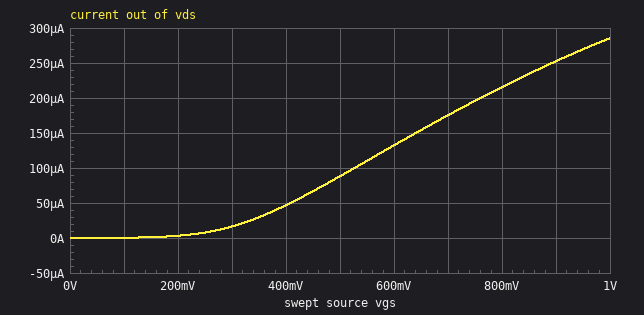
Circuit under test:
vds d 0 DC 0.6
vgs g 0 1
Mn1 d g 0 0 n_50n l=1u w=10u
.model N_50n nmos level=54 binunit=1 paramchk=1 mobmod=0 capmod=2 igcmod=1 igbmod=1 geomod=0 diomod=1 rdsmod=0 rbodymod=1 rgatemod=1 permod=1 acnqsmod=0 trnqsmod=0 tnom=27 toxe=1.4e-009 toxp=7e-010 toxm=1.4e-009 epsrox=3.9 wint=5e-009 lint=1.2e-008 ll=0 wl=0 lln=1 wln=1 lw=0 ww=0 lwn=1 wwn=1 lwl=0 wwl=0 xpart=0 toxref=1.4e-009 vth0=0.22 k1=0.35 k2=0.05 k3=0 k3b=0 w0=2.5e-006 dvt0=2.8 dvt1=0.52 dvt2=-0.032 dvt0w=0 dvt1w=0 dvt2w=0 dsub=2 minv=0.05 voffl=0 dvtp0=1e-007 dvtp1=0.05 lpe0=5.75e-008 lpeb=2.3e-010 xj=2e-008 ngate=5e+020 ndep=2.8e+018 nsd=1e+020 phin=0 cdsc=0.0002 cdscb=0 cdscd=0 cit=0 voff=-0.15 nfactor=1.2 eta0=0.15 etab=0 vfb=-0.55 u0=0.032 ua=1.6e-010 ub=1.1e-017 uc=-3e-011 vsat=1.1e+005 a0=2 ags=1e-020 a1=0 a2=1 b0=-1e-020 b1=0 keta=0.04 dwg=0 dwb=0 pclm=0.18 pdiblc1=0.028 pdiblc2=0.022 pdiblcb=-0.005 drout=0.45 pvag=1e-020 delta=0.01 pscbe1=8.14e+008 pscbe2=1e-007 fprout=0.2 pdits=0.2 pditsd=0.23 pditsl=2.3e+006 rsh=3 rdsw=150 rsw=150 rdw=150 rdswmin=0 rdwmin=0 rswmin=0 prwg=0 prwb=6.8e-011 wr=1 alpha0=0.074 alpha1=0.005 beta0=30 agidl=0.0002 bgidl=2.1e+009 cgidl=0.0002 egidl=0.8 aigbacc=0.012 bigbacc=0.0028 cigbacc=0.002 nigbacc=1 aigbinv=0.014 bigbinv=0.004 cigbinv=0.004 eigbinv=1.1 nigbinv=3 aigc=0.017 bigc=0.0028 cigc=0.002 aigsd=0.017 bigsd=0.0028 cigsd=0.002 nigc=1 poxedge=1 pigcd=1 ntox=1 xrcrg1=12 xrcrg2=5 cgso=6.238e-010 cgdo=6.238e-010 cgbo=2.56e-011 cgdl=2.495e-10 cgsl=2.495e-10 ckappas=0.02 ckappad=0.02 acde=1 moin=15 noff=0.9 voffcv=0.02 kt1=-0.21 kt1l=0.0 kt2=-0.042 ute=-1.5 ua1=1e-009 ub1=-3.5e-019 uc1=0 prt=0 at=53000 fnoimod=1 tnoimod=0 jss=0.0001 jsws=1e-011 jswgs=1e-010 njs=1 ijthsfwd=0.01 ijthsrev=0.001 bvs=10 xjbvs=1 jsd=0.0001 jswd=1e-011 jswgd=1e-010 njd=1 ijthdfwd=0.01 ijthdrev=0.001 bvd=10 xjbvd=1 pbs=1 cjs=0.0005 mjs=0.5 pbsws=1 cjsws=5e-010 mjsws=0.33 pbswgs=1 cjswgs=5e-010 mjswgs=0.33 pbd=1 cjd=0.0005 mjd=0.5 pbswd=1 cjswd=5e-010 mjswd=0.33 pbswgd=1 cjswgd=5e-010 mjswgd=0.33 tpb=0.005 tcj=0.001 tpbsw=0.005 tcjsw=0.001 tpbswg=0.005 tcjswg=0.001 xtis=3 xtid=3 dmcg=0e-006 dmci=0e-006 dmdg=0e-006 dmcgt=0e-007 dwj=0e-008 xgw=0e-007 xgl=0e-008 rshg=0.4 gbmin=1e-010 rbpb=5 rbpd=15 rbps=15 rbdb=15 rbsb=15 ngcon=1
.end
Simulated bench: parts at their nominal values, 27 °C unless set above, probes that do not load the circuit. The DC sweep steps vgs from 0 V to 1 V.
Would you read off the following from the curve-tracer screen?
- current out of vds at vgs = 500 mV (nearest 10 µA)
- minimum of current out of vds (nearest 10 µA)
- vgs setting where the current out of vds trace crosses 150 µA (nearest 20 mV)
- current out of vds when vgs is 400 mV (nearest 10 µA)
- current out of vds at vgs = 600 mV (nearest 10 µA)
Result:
90 µA
0 A
640 mV
50 µA
130 µA
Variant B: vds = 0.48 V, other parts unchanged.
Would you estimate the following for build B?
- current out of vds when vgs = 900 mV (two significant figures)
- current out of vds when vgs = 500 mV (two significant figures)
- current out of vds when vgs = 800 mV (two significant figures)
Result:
250 µA
86 µA
210 µA
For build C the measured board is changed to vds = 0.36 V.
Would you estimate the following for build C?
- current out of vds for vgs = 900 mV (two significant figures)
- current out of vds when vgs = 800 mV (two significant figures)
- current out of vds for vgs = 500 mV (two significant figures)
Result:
230 µA
200 µA
84 µA
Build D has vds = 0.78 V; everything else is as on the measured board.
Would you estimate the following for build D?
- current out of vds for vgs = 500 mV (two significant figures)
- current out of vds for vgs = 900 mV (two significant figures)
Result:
91 µA
260 µA
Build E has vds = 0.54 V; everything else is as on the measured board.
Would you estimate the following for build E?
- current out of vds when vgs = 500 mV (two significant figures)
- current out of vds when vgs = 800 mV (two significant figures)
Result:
87 µA
210 µA
